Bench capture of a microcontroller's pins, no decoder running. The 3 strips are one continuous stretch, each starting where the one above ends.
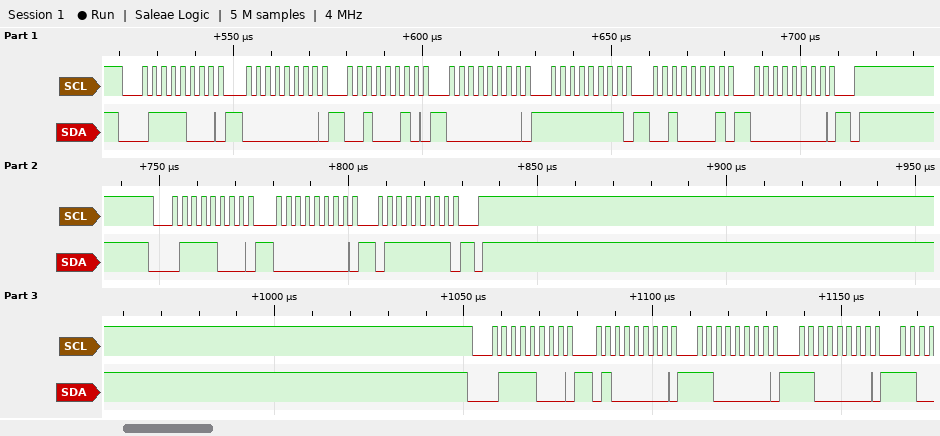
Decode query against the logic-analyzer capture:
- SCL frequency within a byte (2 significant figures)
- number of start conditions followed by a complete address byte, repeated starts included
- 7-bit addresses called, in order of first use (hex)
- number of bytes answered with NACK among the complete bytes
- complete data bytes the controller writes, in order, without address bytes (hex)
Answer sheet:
400 kHz
3
0x3C
0
00 22 00 FF 21 00 00 7F 40 C0 C0
